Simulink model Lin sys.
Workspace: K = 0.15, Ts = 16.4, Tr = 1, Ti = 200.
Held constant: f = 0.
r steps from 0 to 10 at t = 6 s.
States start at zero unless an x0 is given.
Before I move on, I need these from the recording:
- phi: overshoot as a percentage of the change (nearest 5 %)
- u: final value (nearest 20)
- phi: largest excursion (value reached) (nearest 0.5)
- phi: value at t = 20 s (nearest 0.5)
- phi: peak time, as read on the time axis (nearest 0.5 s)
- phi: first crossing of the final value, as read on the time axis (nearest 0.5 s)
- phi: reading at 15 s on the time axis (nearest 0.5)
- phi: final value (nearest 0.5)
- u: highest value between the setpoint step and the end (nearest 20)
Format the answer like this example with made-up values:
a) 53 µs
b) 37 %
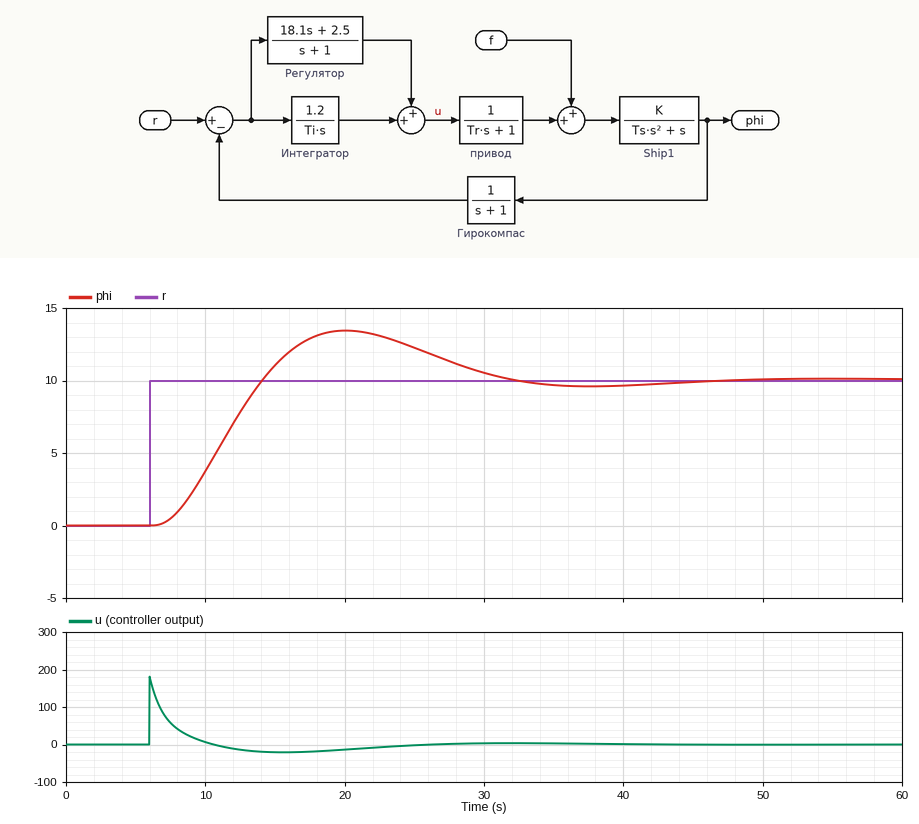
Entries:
a) 35 %
b) 0
c) 13.5
d) 13.5
e) 20.0 s
f) 14.0 s
g) 11.0
h) 10.0
i) 180
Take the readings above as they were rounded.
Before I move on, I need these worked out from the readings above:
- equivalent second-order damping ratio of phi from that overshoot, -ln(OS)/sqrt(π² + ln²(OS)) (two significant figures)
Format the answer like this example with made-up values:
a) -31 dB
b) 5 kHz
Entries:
a) 0.32
